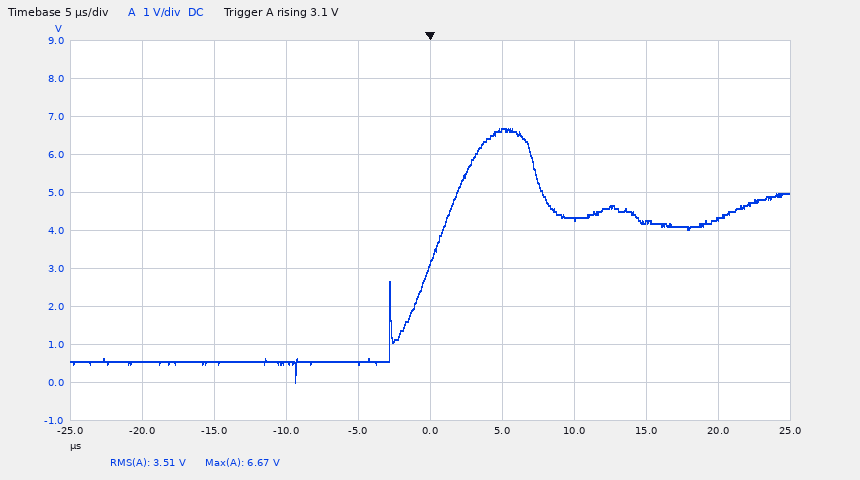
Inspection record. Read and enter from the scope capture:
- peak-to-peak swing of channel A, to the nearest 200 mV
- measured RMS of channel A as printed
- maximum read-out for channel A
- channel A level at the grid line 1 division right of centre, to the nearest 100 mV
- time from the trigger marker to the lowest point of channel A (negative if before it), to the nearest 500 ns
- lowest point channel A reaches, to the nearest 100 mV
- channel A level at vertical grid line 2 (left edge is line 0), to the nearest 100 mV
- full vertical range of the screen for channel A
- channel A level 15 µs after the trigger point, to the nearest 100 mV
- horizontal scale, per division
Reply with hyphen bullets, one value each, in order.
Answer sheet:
- 6.6 V
- 3.51 V
- 6.67 V
- 6.6 V
- -9.5 µs
- 0.0 V
- 600 mV
- 10 V
- 4.2 V
- 5 µs
